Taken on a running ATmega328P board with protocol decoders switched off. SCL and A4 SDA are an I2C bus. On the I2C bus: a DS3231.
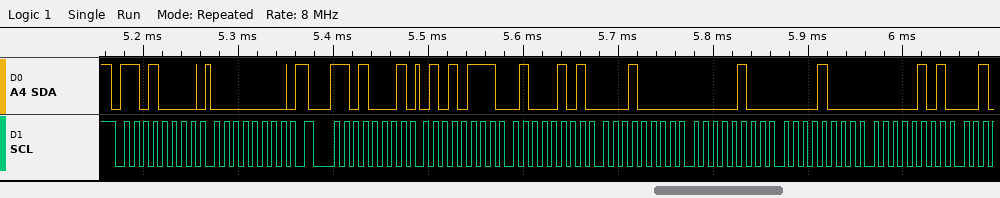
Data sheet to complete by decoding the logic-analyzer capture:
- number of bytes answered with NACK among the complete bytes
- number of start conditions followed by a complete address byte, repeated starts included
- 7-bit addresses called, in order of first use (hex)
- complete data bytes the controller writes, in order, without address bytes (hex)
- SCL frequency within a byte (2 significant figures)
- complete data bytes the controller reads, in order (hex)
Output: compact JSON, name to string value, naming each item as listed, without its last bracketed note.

{"number of bytes answered with NACK among the complete bytes": "0", "number of start conditions followed by a complete address byte, repeated starts included": "2", "7-bit addresses called, in order of first use": "0x68", "complete data bytes the controller writes, in order, without address bytes": "00", "SCL frequency within a byte": "100 kHz", "complete data bytes the controller reads, in order": "57 45 10 04 08 05"}
